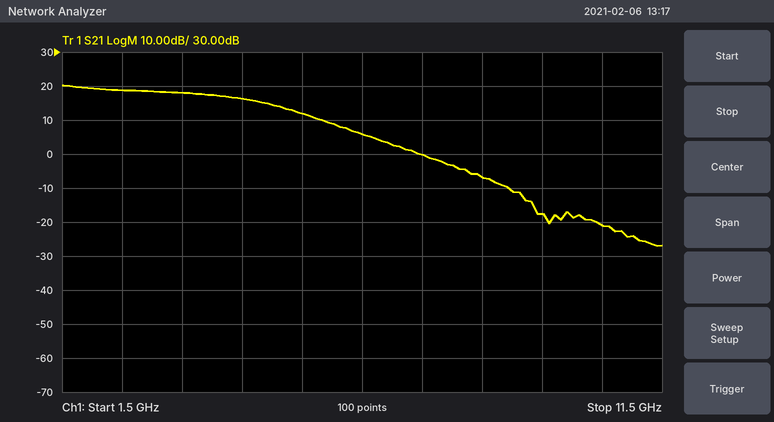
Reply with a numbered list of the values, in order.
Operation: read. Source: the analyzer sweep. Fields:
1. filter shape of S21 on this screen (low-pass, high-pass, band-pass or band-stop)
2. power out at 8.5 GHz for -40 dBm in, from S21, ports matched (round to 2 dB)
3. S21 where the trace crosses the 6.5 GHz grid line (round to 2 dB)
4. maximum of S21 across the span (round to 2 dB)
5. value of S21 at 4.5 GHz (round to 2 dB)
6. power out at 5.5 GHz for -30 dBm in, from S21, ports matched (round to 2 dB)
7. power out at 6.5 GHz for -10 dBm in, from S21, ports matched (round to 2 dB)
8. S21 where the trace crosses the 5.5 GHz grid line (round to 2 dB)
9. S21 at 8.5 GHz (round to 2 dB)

1. low-pass
2. -46 dBm
3. 6 dB
4. 20 dB
5. 16 dB
6. -18 dBm
7. -4 dBm
8. 12 dB
9. -6 dB
